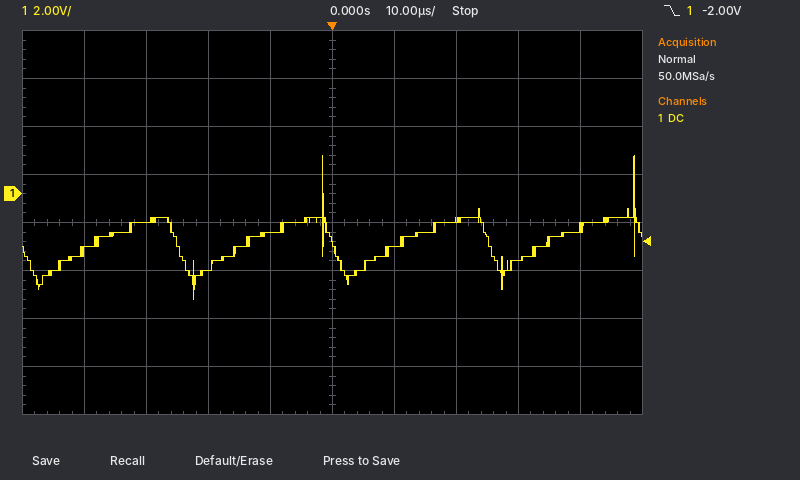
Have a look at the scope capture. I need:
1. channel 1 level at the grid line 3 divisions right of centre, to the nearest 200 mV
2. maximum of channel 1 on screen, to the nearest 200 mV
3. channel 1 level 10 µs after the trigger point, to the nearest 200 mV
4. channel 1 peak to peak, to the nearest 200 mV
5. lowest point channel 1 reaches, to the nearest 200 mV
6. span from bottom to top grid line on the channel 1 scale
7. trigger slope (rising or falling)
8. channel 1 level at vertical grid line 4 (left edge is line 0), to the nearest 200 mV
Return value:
-2.8 V
1.6 V
-2.2 V
6.0 V
-4.4 V
16 V
falling
-1.6 V
